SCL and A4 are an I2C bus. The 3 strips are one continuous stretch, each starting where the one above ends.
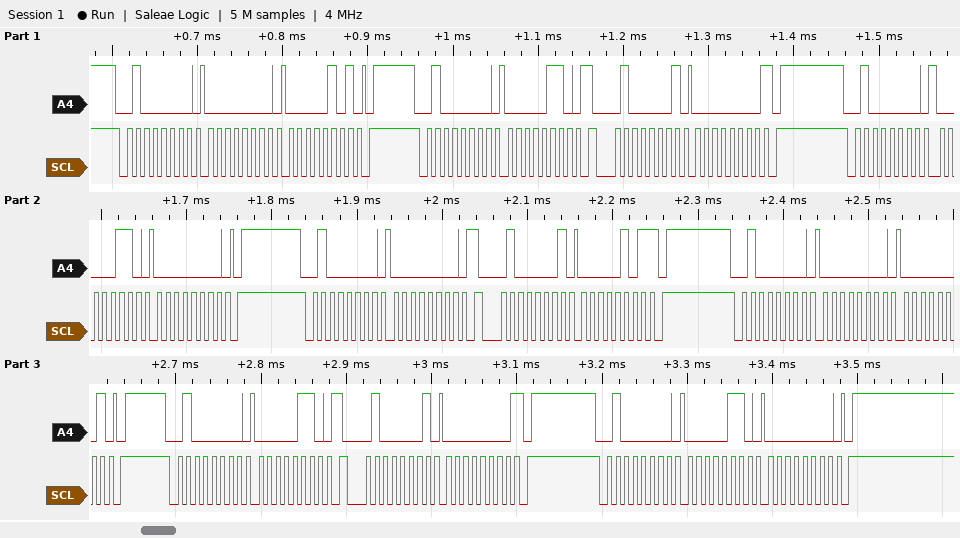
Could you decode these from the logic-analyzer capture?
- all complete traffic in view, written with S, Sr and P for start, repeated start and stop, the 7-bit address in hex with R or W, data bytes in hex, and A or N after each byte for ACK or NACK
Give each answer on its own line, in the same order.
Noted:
S 20W A 00 A 05 A P S 20W A 06 A Sr 20R A 00 N P S 20W A 06 A 00 A P S 20W A 00 A Sr 20R A 05 N P S 20W A 00 A 01 A P S 20W A 06 A Sr 20R A 00 N P S 20W A 06 A 00 A P
